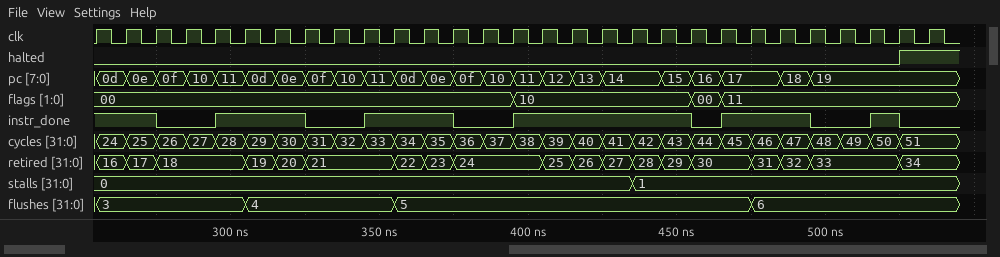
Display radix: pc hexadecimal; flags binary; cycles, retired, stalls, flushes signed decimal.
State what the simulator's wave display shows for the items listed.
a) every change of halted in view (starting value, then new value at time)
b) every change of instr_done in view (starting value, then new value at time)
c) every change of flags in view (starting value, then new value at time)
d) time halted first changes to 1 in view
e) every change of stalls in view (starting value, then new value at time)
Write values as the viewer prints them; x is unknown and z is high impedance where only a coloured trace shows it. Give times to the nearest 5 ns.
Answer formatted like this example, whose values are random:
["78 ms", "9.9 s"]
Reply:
["0, 1 at 525 ns", "1, 0 at 275 ns, 1 at 295 ns, 0 at 325 ns, 1 at 345 ns, 0 at 375 ns, 1 at 395 ns, 0 at 455 ns, 1 at 465 ns, 0 at 495 ns, 1 at 515 ns, 0 at 525 ns", "00, 10 at 395 ns, 00 at 455 ns, 11 at 465 ns", "525 ns", "0, 1 at 435 ns"]
